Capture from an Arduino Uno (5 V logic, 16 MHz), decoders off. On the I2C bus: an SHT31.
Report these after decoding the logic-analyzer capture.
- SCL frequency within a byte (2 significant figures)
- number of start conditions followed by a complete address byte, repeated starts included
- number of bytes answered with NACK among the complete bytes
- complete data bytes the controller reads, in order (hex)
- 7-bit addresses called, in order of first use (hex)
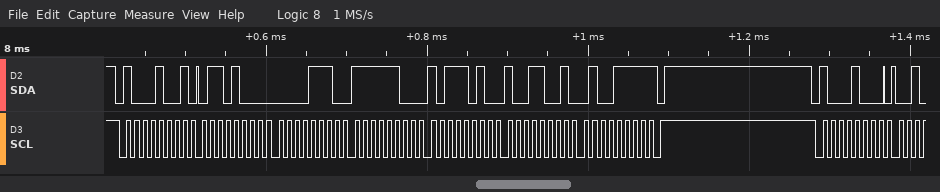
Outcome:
100 kHz
2
1
68 0E FC BA 99 4F
0x44
